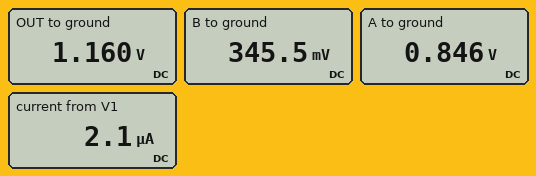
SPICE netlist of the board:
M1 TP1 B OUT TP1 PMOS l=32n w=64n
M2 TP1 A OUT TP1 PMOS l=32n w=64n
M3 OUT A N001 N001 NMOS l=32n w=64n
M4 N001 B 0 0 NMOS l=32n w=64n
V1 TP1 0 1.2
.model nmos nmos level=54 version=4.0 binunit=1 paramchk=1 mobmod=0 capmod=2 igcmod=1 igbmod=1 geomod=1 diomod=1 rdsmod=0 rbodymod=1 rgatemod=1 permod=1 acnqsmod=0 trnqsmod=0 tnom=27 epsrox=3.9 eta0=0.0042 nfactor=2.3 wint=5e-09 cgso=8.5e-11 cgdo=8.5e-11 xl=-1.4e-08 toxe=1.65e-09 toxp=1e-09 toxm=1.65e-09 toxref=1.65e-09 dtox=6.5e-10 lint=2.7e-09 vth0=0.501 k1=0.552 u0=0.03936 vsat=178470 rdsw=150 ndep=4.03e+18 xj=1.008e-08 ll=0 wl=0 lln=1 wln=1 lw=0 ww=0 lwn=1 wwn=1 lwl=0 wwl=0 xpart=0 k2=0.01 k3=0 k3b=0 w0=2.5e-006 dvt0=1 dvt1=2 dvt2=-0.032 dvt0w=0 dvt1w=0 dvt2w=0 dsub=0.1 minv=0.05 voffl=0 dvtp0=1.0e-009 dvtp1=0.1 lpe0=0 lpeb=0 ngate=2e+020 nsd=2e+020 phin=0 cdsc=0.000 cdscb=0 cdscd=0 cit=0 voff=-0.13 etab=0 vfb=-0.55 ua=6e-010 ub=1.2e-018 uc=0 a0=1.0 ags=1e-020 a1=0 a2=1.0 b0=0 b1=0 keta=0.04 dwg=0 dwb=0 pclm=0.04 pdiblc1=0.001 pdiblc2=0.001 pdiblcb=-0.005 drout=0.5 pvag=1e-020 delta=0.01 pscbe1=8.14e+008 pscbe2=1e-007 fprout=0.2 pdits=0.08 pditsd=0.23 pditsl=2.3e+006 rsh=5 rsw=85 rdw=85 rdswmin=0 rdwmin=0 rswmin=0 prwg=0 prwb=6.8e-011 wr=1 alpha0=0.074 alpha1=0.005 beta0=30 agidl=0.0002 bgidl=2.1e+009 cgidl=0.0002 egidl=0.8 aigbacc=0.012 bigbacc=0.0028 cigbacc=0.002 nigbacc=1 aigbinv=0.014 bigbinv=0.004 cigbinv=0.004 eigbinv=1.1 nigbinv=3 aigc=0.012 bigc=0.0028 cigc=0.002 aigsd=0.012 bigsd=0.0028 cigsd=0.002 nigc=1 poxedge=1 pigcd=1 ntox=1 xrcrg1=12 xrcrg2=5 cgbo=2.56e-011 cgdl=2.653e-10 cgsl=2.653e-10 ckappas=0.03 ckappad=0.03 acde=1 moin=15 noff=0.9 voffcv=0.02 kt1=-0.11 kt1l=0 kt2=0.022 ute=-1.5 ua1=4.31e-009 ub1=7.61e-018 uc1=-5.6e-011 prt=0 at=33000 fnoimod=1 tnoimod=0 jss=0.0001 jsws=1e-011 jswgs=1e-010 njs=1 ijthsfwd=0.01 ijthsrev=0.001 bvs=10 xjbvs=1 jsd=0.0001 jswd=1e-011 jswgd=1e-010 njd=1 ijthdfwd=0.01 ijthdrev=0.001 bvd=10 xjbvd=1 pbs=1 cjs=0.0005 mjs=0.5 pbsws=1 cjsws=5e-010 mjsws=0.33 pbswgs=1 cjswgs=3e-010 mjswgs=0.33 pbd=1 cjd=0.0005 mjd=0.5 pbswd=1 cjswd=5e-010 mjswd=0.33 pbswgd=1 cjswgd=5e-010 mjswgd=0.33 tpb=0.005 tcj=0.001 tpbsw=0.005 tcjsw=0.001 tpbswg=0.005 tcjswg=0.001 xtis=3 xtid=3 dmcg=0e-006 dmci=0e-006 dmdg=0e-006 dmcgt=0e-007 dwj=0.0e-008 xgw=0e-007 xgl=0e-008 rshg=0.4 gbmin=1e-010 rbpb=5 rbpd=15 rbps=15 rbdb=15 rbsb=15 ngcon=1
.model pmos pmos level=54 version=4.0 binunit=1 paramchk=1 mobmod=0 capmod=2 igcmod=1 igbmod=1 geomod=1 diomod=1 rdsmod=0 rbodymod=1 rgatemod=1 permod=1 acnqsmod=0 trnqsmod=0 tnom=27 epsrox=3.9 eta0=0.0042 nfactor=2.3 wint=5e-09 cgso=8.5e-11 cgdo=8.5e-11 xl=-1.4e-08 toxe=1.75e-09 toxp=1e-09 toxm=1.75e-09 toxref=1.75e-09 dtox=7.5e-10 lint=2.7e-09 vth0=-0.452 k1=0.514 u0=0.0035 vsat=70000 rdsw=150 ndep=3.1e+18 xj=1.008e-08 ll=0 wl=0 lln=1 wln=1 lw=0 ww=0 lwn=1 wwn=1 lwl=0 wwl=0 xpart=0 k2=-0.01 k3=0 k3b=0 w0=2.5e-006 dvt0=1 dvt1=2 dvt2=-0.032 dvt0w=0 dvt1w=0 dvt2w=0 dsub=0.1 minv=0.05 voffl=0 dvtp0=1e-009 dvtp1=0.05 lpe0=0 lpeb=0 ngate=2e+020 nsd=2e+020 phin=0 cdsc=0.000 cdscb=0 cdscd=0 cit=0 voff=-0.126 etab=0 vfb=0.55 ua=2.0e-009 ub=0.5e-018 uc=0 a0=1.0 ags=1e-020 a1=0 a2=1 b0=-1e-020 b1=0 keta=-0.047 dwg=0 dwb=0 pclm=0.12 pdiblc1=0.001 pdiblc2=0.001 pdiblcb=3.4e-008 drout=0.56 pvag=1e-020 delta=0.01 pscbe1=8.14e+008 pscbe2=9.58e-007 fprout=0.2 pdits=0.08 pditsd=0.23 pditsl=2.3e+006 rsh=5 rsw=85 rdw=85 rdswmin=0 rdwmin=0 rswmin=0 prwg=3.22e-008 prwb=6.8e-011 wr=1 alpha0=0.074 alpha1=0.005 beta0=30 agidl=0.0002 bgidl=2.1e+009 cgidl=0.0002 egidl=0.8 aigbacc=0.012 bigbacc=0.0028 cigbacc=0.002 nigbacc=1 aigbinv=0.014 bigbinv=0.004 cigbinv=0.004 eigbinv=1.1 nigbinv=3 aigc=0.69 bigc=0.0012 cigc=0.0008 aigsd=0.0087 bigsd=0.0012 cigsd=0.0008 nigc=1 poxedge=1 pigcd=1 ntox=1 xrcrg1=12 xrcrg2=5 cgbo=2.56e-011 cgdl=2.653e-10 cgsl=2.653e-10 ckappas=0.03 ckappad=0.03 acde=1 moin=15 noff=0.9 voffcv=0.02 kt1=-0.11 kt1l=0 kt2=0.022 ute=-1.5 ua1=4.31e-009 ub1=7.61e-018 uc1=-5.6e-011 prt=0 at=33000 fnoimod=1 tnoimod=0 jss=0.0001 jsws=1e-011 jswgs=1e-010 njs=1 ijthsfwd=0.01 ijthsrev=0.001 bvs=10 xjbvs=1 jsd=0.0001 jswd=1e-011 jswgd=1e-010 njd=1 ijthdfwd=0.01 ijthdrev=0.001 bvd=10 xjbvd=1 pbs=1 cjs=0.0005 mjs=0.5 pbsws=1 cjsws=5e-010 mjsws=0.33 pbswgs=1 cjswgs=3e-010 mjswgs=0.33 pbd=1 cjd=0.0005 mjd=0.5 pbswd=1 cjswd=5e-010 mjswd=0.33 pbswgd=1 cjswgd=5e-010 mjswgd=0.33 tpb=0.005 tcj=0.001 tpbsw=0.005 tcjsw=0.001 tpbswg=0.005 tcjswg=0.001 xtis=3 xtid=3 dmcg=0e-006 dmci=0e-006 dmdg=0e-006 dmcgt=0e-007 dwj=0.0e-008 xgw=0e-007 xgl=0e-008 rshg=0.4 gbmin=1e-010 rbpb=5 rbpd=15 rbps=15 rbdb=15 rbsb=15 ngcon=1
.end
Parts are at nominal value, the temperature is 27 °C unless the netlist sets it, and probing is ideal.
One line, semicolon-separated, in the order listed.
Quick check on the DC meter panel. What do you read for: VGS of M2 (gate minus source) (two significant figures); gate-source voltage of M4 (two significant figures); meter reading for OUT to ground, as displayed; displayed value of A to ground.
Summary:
-310 mV; 350 mV; 1.160 V; 0.846 V
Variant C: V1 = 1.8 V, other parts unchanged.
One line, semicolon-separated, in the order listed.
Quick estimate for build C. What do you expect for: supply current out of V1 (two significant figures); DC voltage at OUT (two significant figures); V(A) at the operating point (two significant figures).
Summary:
21 µA; 1.6 V; 1.1 V
